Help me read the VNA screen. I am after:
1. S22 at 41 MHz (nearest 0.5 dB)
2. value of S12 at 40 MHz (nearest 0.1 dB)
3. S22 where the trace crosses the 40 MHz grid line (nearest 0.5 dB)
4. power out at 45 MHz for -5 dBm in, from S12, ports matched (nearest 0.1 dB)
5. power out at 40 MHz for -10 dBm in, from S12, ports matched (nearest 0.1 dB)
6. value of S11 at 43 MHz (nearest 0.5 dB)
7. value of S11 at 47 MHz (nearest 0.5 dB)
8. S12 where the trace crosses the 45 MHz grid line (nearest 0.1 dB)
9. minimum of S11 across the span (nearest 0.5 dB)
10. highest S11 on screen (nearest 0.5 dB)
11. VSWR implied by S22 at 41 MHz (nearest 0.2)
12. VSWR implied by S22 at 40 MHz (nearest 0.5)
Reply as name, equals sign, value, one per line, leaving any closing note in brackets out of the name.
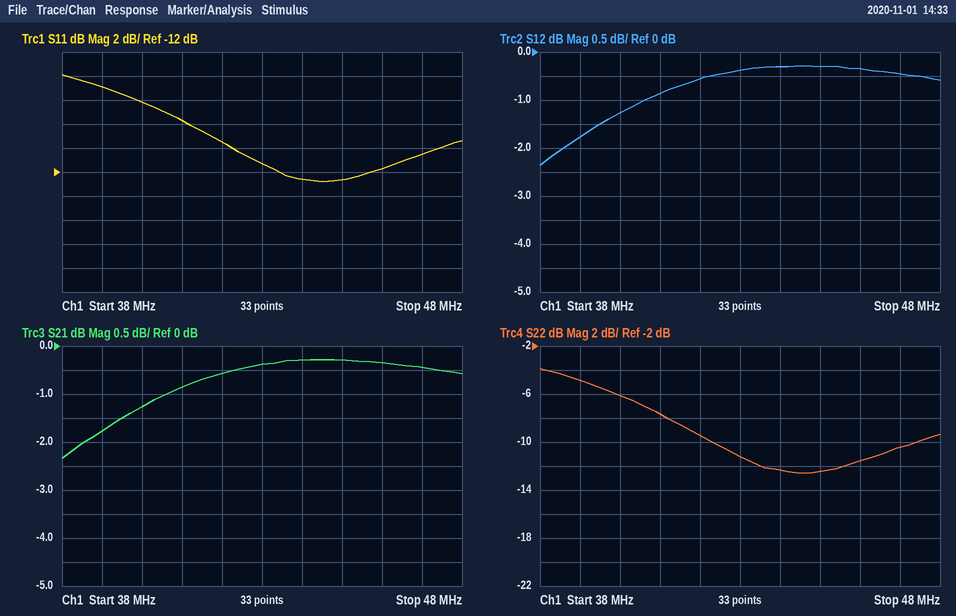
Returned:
S22 at 41 MHz = -7.5 dB
value of S12 at 40 MHz = -1.3 dB
S22 where the trace crosses the 40 MHz grid line = -6.0 dB
power out at 45 MHz for -5 dBm in, from S12, ports matched = -5.3 dBm
power out at 40 MHz for -10 dBm in, from S12, ports matched = -11.3 dBm
value of S11 at 43 MHz = -11.5 dB
value of S11 at 47 MHz = -10.5 dB
S12 where the trace crosses the 45 MHz grid line = -0.3 dB
minimum of S11 across the span = -13.0 dB
highest S11 on screen = -4.0 dB
VSWR implied by S22 at 41 MHz = 2.4
VSWR implied by S22 at 40 MHz = 3.0
